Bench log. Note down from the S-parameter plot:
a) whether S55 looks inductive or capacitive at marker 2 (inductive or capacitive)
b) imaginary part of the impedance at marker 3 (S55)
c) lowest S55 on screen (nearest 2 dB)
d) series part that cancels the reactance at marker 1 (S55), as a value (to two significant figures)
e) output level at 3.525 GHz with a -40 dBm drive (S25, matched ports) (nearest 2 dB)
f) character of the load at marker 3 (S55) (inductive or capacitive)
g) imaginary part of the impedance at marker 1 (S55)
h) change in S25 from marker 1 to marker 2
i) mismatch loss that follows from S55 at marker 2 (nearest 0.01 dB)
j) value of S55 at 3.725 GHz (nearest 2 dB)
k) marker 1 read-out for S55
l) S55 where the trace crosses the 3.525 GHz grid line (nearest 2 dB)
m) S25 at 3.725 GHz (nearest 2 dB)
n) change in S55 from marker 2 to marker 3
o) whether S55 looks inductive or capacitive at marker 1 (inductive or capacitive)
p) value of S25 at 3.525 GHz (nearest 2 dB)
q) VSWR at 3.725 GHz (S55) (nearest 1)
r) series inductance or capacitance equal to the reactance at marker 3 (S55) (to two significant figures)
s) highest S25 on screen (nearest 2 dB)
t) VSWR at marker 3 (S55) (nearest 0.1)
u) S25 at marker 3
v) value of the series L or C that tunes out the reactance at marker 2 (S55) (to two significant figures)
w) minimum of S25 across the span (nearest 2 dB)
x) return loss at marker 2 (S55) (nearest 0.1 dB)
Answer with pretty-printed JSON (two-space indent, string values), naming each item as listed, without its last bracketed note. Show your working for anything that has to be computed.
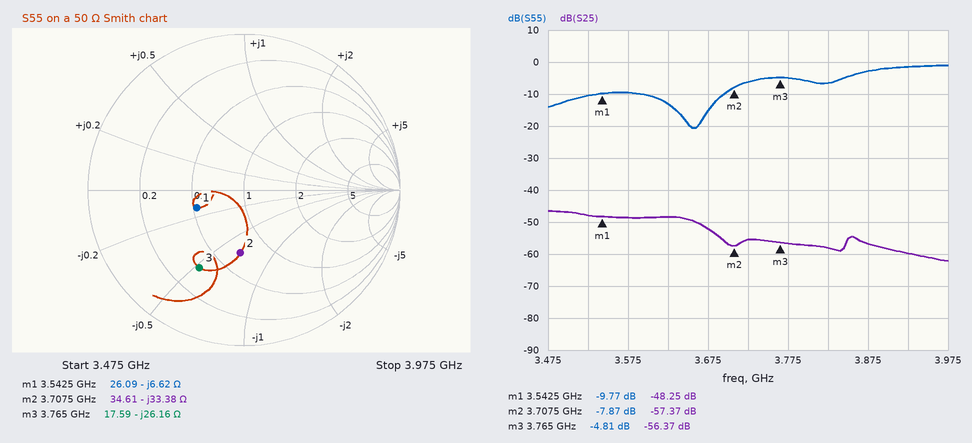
{
  "whether S55 looks inductive or capacitive at marker 2": "capacitive",
  "imaginary part of the impedance at marker 3": "-26.16 Ω",
  "lowest S55 on screen": "-20 dB",
  "series part that cancels the reactance at marker 1 (S55), as a value": "L = 6.62 Ω/(2π × 3.5425 GHz) ≈ 297 pH, so 300 pH to two significant figures",
  "output level at 3.525 GHz with a -40 dBm drive (S25, matched ports)": "-40 dBm + (-48 dB) = -88 dBm",
  "character of the load at marker 3 (S55)": "capacitive",
  "imaginary part of the impedance at marker 1": "-6.62 Ω",
  "change in S25 from marker 1 to marker 2": "-57.37 − (-48.25) = -9.12 dB",
  "mismatch loss that follows from S55 at marker 2": "−10 log10(1 − 10^(-7.87/10)) ≈ 0.77 dB",
  "value of S55 at 3.725 GHz": "-6 dB",
  "marker 1 read-out for S55": "-9.77 dB",
  "S55 where the trace crosses the 3.525 GHz grid line": "-10 dB",
  "S25 at 3.725 GHz": "-56 dB",
  "change in S55 from marker 2 to marker 3": "-4.81 − (-7.87) = 3.06 dB",
  "whether S55 looks inductive or capacitive at marker 1": "capacitive",
  "value of S25 at 3.525 GHz": "-48 dB",
  "VSWR at 3.725 GHz (S55)": "|Γ| = 10^(-6/20) = 0.5012; VSWR = (1 + 0.5012)/(1 − 0.5012) ≈ 3",
  "series inductance or capacitance equal to the reactance at marker 3 (S55)": "C = 1/(2π × 3.765 GHz × 26.16 Ω) ≈ 1.6 pF",
  "highest S25 on screen": "-46 dB",
  "VSWR at marker 3 (S55)": "3.7",
  "S25 at marker 3": "-56.37 dB",
  "value of the series L or C that tunes out the reactance at marker 2 (S55)": "L = 33.38 Ω/(2π × 3.7075 GHz) ≈ 1.4 nH",
  "minimum of S25 across the span": "-62 dB",
  "return loss at marker 2 (S55)": "7.9 dB"
}
